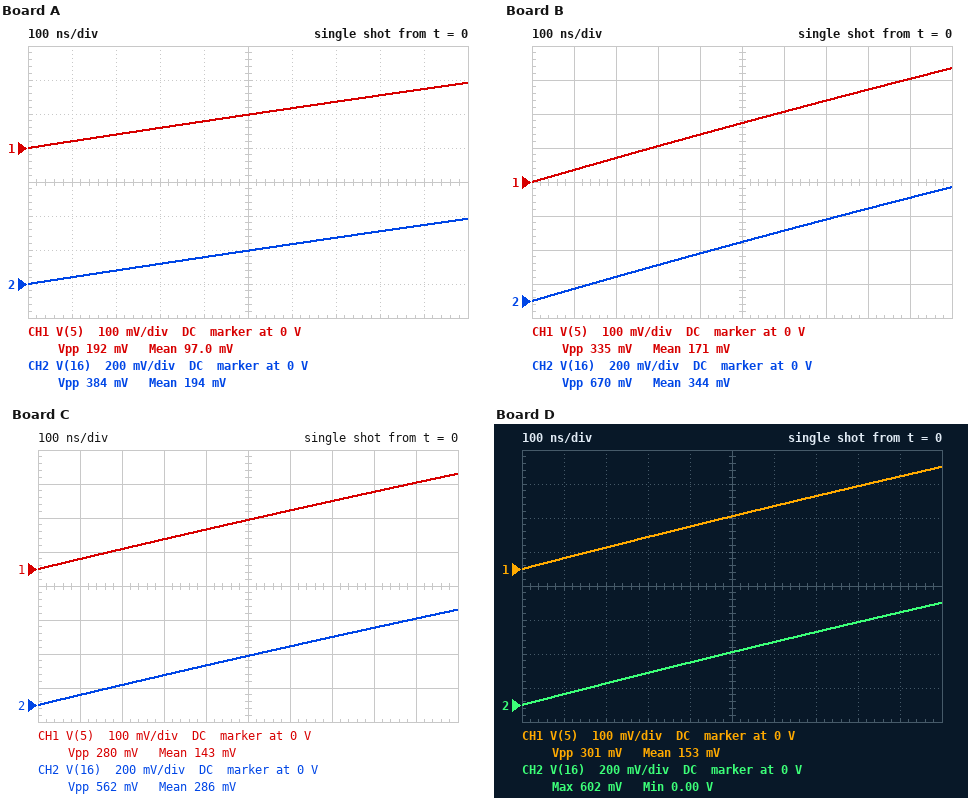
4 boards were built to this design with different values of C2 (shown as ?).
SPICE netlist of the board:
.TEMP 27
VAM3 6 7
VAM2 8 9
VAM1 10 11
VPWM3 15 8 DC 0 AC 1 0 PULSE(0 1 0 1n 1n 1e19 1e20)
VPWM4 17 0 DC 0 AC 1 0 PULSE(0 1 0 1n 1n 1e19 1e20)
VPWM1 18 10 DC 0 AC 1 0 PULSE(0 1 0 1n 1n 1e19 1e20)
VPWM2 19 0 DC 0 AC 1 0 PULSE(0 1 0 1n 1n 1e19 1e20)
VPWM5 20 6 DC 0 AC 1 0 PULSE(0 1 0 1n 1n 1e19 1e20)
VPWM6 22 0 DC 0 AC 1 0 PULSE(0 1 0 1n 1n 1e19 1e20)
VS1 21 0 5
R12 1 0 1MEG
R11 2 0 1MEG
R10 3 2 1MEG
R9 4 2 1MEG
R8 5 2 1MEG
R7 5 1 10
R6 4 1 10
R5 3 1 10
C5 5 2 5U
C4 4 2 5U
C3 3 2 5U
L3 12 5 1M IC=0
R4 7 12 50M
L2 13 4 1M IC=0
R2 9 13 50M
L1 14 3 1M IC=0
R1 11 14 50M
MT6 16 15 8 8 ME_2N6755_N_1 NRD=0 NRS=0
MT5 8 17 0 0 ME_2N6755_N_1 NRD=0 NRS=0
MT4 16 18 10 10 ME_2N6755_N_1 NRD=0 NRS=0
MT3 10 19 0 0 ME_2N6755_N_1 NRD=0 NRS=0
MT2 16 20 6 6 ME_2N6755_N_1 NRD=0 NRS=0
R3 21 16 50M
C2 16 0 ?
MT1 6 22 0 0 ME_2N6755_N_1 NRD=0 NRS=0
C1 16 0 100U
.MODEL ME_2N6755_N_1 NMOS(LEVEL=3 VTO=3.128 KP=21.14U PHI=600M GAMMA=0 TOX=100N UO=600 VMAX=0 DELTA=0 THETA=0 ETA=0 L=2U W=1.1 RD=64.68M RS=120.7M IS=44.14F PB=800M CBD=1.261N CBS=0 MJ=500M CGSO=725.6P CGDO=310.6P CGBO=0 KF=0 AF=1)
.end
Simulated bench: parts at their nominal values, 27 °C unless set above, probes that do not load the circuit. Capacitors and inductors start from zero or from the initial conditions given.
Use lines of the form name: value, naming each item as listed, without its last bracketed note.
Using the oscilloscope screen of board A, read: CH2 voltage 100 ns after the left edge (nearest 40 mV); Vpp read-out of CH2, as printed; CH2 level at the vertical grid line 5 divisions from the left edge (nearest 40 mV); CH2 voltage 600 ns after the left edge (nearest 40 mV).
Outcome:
CH2 voltage 100 ns after the left edge: 40 mV
Vpp read-out of CH2, as printed: 384 mV
CH2 level at the vertical grid line 5 divisions from the left edge: 200 mV
CH2 voltage 600 ns after the left edge: 240 mV
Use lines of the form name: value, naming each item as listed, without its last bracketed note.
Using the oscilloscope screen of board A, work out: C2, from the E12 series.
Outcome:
C2, from the E12 series: 150 µF
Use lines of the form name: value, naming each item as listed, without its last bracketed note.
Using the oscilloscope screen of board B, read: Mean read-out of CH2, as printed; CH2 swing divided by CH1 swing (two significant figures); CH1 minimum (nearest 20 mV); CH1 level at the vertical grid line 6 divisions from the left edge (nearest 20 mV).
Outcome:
Mean read-out of CH2, as printed: 344 mV
CH2 swing divided by CH1 swing: 2.0
CH1 minimum: 0 V
CH1 level at the vertical grid line 6 divisions from the left edge: 200 mV
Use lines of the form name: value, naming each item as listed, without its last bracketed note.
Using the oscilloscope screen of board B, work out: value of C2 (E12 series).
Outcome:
value of C2: 39 µF
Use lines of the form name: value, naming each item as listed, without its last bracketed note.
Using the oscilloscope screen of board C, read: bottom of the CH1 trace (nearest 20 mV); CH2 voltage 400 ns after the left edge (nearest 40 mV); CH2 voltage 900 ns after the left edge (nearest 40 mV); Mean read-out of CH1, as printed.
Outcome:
bottom of the CH1 trace: 0 V
CH2 voltage 400 ns after the left edge: 240 mV
CH2 voltage 900 ns after the left edge: 520 mV
Mean read-out of CH1, as printed: 143 mV
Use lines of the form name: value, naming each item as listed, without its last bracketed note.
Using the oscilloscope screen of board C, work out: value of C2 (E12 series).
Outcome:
value of C2: 68 µF
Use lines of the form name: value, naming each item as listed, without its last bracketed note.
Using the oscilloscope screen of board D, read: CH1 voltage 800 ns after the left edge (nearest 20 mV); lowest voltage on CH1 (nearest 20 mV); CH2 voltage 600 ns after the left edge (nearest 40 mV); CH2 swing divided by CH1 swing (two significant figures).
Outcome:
CH1 voltage 800 ns after the left edge: 240 mV
lowest voltage on CH1: 0 V
CH2 voltage 600 ns after the left edge: 360 mV
CH2 swing divided by CH1 swing: 2.0
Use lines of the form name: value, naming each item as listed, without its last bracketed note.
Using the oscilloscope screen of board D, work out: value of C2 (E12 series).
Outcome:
value of C2: 56 µF
